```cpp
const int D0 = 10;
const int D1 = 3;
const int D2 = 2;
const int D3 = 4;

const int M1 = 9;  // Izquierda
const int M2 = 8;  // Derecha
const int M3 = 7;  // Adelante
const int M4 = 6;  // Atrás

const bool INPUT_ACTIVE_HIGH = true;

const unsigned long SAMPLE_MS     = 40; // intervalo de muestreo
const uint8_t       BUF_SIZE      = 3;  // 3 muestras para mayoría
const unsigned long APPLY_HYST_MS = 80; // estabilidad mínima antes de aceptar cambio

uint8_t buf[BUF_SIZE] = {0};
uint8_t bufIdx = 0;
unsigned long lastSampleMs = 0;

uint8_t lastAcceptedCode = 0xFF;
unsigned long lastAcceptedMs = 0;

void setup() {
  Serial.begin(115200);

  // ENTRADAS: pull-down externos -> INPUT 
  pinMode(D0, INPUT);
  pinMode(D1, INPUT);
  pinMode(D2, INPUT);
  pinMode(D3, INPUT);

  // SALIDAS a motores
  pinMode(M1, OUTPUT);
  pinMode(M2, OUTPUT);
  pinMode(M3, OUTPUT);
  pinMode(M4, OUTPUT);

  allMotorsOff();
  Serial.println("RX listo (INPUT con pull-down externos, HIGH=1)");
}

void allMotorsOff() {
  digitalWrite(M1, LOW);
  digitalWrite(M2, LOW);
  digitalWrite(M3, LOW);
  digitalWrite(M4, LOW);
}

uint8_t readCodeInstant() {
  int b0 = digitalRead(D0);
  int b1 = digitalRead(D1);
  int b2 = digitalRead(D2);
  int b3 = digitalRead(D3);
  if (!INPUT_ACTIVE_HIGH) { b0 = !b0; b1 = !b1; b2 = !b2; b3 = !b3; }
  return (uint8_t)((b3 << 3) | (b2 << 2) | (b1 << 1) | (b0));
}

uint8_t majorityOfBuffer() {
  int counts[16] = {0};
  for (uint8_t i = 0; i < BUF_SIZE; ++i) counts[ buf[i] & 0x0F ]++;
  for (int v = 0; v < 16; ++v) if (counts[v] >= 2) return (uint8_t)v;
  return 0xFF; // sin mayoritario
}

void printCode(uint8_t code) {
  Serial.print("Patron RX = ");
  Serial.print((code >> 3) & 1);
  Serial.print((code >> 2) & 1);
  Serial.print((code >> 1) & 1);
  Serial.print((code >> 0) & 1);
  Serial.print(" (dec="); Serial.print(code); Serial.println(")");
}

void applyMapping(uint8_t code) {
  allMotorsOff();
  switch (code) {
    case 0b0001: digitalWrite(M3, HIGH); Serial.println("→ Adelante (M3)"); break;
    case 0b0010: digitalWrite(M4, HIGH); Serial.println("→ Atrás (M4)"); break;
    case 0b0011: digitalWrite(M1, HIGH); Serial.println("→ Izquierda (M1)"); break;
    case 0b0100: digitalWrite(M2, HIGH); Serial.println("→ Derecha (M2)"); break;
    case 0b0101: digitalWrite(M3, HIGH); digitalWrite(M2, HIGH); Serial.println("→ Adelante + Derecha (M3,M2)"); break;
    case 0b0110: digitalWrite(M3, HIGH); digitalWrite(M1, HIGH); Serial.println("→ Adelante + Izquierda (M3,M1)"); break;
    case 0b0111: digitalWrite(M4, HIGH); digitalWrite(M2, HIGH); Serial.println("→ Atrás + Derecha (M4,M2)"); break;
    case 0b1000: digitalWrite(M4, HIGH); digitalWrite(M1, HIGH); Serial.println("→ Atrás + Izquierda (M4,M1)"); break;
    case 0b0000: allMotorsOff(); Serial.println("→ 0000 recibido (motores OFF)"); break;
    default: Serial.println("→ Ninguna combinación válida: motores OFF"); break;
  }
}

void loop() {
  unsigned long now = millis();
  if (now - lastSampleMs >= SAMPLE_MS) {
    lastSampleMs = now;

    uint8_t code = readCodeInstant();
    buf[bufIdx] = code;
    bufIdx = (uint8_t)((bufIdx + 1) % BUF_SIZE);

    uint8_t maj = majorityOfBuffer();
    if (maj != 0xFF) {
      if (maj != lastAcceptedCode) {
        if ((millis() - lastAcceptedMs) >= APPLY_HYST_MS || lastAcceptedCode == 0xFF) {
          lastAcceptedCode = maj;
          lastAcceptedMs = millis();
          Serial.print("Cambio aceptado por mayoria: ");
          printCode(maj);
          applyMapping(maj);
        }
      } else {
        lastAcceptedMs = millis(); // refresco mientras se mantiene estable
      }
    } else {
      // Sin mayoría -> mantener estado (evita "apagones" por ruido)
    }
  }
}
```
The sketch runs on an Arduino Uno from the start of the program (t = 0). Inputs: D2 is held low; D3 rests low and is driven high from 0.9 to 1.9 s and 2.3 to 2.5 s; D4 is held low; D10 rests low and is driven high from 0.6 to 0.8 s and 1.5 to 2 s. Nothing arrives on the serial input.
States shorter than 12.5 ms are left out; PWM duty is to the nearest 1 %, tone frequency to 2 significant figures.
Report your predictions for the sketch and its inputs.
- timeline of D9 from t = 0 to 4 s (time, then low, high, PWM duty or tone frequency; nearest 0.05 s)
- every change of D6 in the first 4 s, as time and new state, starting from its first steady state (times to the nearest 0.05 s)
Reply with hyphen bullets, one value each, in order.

- 0 s low; 1.6 s high; 2 s low
- 0 s low; 1 s high; 1.6 s low; 2.4 s high; 2.6 s low
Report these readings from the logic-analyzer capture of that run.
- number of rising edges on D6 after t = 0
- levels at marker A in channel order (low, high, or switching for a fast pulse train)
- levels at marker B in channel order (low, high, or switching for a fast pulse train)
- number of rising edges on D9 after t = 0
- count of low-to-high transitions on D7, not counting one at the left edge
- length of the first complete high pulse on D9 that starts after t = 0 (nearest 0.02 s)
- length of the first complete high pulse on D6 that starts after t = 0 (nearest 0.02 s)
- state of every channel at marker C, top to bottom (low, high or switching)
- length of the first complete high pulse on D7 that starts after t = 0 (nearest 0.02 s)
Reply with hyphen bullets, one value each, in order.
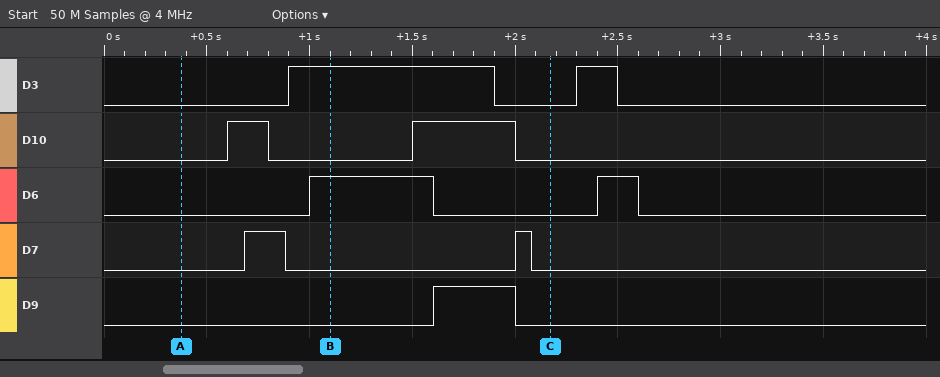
- 2
- D3 low, D10 low, D6 low, D7 low, D9 low
- D3 high, D10 low, D6 high, D7 low, D9 low
- 1
- 2
- 0.40 s
- 0.60 s
- D3 low, D10 low, D6 low, D7 low, D9 low
- 0.20 s
